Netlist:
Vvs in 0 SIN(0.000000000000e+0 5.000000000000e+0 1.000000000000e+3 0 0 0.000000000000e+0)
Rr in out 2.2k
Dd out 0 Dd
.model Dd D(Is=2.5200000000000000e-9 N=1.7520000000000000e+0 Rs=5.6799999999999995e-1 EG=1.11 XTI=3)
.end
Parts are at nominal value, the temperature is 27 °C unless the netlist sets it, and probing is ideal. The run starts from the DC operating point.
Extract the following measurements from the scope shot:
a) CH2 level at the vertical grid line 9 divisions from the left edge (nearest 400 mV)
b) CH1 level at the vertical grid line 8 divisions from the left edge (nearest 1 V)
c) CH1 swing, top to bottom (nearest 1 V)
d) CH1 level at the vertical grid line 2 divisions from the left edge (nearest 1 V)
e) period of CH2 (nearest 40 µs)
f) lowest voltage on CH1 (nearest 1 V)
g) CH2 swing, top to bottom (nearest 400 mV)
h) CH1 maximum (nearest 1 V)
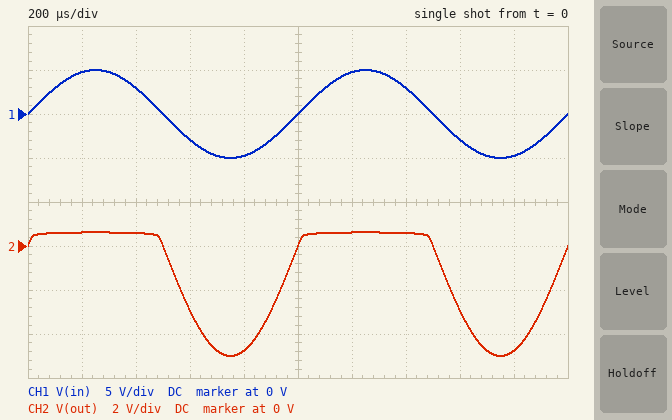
-4.8 V
-3 V
10 V
3 V
1.00 ms
-5 V
5.6 V
5 V
